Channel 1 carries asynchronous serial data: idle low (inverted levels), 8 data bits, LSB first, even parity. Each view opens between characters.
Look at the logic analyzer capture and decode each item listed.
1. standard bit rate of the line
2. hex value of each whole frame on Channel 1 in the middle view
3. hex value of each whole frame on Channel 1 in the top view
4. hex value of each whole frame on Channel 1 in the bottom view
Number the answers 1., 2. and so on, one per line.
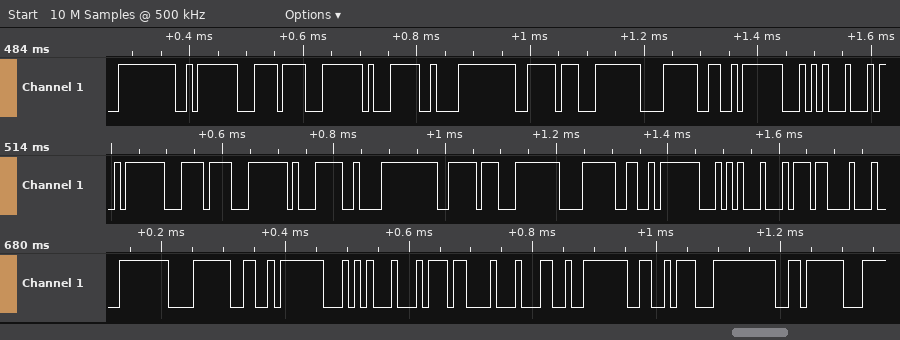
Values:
1. 100000 baud
2. 01, 08, 40, B0, 00, 10, 80, 60, 01, 75, 91
3. 00, 01, 08, 40, B0, 00, 10, 80, 60, 01, 75
4. 80, 60, 01, 75, 91, 77, 03, 16, 00, 02
